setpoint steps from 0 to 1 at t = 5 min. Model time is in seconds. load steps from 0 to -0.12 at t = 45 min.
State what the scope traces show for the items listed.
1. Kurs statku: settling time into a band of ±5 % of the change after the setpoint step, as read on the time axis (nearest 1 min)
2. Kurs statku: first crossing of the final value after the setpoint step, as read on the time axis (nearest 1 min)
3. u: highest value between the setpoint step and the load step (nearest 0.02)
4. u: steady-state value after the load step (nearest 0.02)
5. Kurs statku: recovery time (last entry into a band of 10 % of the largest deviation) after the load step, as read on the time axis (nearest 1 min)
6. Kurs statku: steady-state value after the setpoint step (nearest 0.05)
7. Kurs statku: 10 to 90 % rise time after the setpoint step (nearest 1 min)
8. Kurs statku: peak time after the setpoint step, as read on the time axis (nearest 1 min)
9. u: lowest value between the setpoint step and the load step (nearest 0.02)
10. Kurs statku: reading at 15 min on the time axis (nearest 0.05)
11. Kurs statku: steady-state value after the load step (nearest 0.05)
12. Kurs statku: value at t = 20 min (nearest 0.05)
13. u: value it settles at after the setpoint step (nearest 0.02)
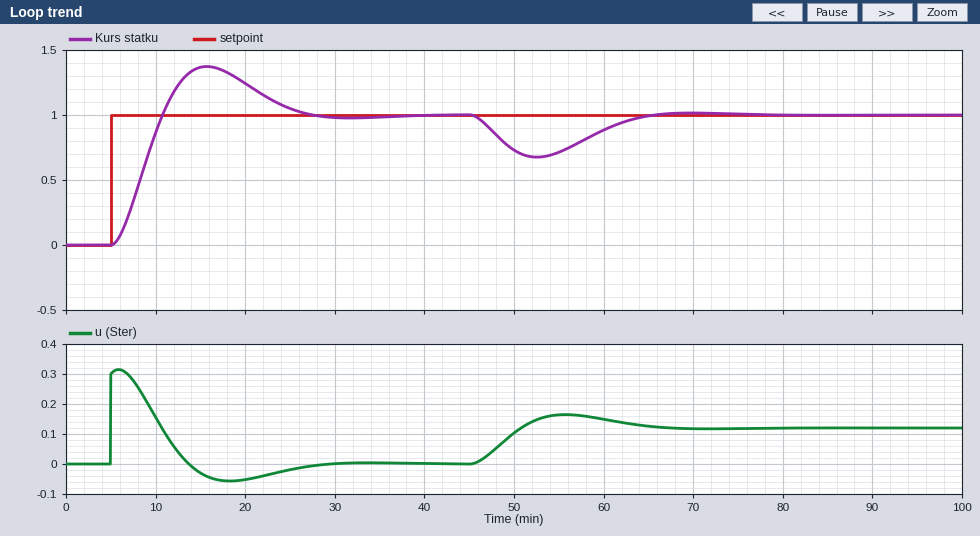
25 min
11 min
0.32
0.12
63 min
1.00
4 min
16 min
-0.06
1.35
1.00
1.25
0.00
